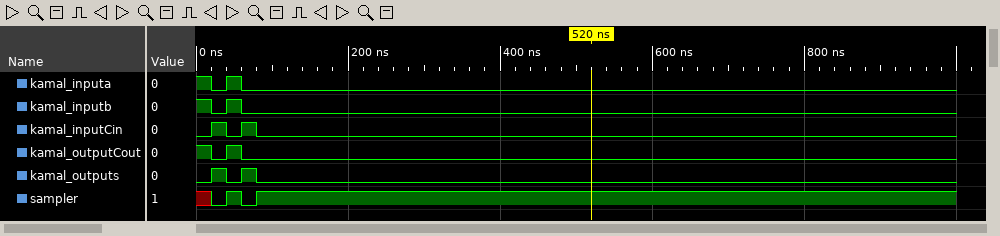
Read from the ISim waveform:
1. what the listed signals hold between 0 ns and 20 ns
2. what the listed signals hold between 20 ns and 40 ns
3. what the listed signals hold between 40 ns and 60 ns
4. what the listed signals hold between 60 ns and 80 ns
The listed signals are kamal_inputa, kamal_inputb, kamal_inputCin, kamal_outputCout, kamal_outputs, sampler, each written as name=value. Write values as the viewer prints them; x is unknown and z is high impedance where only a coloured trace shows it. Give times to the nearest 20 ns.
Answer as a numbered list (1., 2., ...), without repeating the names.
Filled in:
1. kamal_inputa=1, kamal_inputb=1, kamal_inputCin=0, kamal_outputCout=1, kamal_outputs=0, sampler=x
2. kamal_inputa=0, kamal_inputb=0, kamal_inputCin=1, kamal_outputCout=0, kamal_outputs=1, sampler=0
3. kamal_inputa=1, kamal_inputb=1, kamal_inputCin=0, kamal_outputCout=1, kamal_outputs=0, sampler=1
4. kamal_inputa=0, kamal_inputb=0, kamal_inputCin=1, kamal_outputCout=0, kamal_outputs=1, sampler=0
